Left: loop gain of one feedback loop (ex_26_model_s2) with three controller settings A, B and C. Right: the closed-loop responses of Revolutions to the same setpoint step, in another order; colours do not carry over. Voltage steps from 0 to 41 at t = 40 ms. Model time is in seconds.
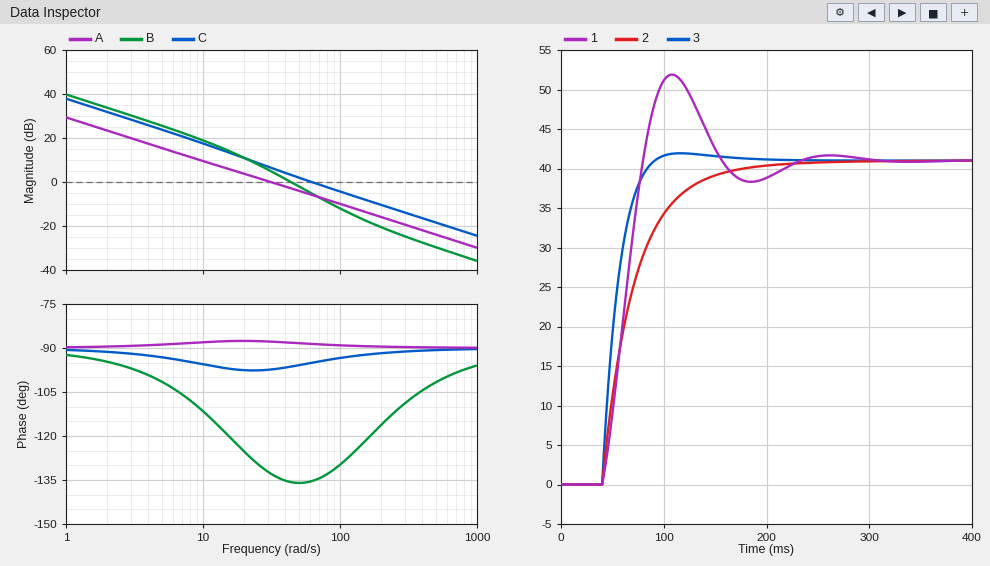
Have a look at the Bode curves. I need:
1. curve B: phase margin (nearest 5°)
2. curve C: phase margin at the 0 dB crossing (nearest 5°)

45°
85°
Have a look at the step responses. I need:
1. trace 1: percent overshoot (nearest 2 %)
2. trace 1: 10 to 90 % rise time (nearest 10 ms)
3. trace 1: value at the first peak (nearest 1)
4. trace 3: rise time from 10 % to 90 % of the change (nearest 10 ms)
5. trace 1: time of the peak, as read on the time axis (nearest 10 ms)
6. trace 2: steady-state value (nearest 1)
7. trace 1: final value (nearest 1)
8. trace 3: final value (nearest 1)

26 %
30 ms
52
30 ms
110 ms
41
41
41
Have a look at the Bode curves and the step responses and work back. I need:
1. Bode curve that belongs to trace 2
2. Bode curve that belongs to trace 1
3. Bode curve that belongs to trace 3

A
B
C
